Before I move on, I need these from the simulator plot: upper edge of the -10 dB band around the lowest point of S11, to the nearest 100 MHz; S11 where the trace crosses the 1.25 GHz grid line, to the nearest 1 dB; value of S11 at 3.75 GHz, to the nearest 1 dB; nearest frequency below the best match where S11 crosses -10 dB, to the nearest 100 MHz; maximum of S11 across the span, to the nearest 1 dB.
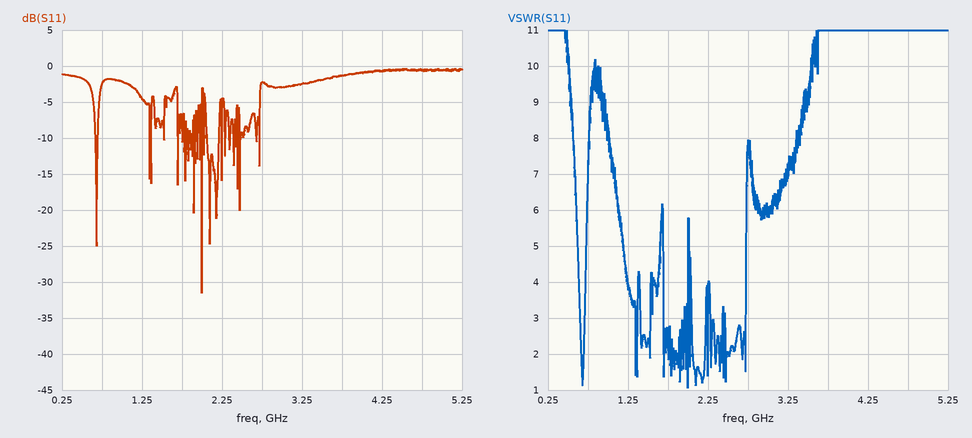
2.0 GHz
-5 dB
-1 dB
2.0 GHz
0 dB
